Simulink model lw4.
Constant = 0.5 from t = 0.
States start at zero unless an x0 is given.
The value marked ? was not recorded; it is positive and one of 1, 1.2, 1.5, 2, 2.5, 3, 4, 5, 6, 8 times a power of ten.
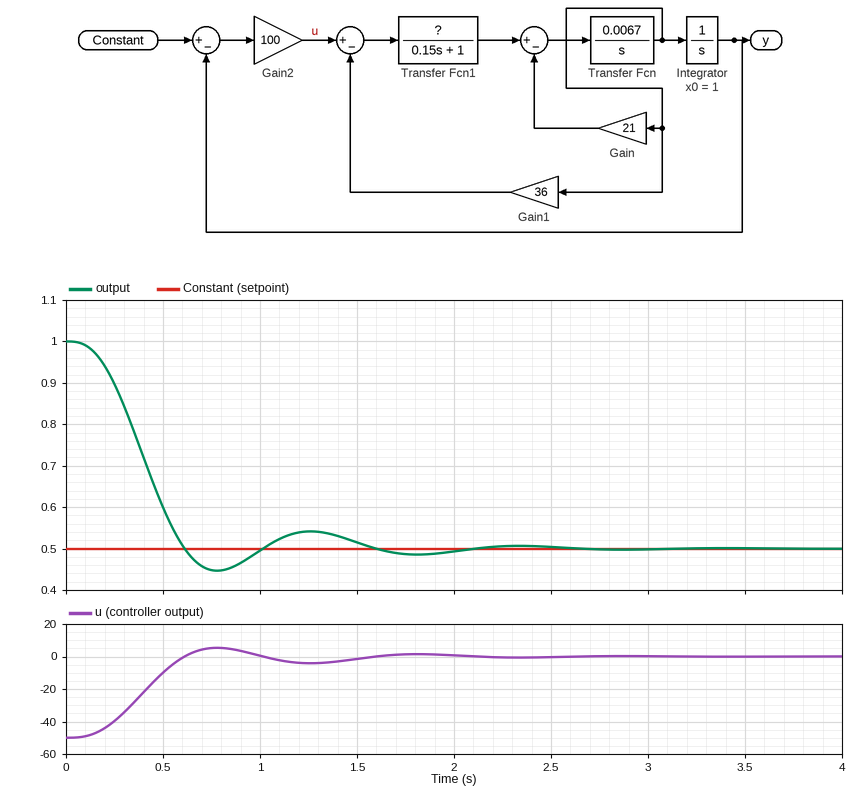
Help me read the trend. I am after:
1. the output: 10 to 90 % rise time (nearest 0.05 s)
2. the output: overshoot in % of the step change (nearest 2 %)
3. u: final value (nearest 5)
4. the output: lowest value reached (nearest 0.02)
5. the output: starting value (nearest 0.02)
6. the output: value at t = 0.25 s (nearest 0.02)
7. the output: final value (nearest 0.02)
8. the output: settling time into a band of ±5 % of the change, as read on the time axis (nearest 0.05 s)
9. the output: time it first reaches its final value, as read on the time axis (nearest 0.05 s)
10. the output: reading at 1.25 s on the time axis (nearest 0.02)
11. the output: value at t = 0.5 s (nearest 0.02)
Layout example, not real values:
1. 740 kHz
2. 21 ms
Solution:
1. 0.35 s
2. 10 %
3. 0
4. 0.44
5. 1.00
6. 0.90
7. 0.50
8. 1.45 s
9. 0.60 s
10. 0.54
11. 0.60
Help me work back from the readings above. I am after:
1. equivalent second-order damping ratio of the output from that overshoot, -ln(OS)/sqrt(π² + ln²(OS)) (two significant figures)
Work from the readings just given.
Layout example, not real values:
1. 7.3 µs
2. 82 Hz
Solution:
1. 0.59
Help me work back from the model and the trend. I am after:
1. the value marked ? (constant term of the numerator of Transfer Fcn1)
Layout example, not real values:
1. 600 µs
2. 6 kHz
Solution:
1. 30
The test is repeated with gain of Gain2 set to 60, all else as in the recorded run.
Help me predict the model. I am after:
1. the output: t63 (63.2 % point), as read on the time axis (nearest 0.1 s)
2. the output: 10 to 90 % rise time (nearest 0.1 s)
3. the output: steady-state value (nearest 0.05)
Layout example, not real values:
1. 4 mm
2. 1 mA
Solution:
1. 0.6 s
2. 1.0 s
3. 0.50
